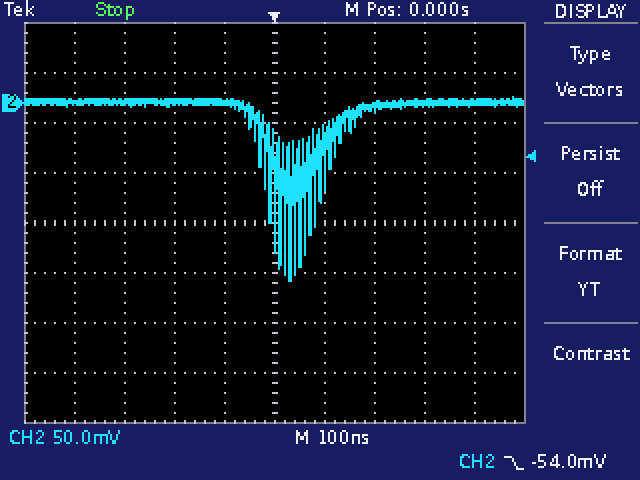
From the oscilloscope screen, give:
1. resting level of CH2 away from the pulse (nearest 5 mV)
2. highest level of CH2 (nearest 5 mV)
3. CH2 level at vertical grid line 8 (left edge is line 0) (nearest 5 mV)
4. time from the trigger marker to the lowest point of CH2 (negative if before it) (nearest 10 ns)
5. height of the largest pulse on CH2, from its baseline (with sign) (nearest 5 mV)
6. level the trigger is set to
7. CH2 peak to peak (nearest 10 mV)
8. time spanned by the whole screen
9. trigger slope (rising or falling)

0 mV
5 mV
0 mV
+30 ns
-180 mV
-54.0 mV
180 mV
1 µs
falling
